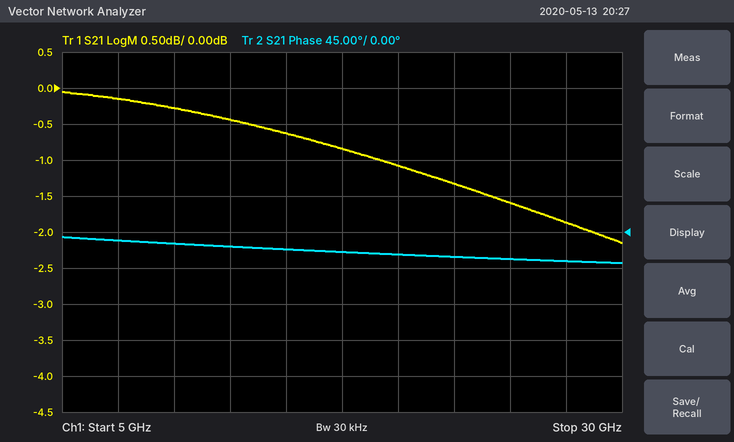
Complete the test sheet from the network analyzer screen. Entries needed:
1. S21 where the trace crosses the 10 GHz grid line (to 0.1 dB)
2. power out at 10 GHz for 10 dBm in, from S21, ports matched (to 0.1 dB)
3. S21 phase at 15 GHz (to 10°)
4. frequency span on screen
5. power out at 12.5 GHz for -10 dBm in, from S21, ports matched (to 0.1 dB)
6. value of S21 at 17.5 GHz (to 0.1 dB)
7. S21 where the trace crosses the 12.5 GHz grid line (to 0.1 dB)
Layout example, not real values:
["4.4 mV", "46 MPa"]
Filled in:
["-0.3 dB", "9.7 dBm", "-20°", "25 GHz", "-10.4 dBm", "-0.8 dB", "-0.4 dB"]
